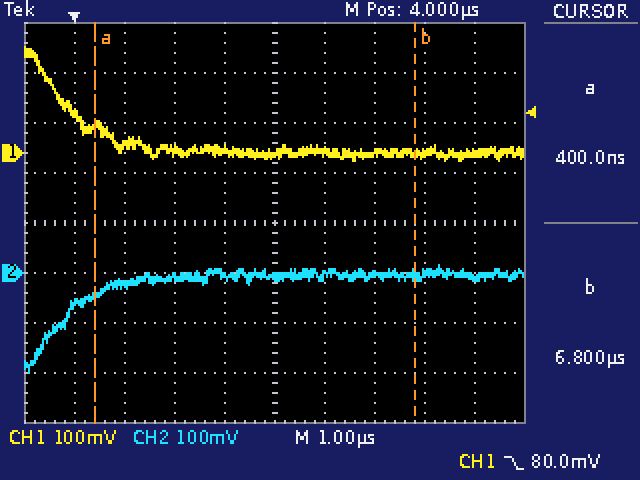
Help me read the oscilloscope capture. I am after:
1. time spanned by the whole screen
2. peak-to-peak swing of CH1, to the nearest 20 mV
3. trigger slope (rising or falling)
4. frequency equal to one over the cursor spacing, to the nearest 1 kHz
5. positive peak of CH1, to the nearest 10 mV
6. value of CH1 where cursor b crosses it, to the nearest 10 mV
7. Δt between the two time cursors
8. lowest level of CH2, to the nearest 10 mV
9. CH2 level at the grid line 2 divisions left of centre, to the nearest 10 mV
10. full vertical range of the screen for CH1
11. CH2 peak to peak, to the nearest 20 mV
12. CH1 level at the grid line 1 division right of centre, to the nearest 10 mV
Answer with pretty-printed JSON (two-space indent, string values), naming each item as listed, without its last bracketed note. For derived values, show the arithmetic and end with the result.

{
  "time spanned by the whole screen": "10 µs",
  "peak-to-peak swing of CH1, to the nearest 20 mV": "220 mV",
  "trigger slope": "falling",
  "frequency equal to one over the cursor spacing, to the nearest 1 kHz": "1 / 6.4 µs ≈ 156 kHz",
  "positive peak of CH1, to the nearest 10 mV": "210 mV",
  "value of CH1 where cursor b crosses it, to the nearest 10 mV": "0 mV",
  "Δt between the two time cursors": "6.8 µs − (400 ns) = 6.4 µs",
  "lowest level of CH2, to the nearest 10 mV": "-200 mV",
  "CH2 level at the grid line 2 divisions left of centre, to the nearest 10 mV": "-10 mV",
  "full vertical range of the screen for CH1": "800 mV",
  "CH2 peak to peak, to the nearest 20 mV": "220 mV",
  "CH1 level at the grid line 1 division right of centre, to the nearest 10 mV": "0 mV"
}
